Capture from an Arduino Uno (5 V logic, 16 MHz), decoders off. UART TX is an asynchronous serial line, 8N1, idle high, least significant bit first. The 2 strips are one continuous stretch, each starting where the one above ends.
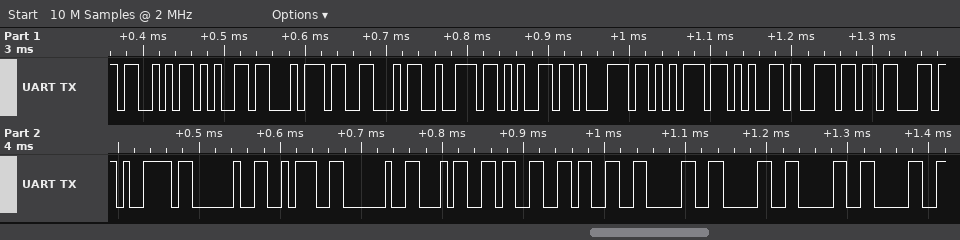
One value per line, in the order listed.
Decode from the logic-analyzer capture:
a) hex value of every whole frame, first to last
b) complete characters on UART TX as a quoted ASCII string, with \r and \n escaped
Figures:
53 65 74 46 72 65 71 75 65 6E 63 79 20 3A 20 34 33 33 30 30 30 30
"SetFrequency : 4330000"
